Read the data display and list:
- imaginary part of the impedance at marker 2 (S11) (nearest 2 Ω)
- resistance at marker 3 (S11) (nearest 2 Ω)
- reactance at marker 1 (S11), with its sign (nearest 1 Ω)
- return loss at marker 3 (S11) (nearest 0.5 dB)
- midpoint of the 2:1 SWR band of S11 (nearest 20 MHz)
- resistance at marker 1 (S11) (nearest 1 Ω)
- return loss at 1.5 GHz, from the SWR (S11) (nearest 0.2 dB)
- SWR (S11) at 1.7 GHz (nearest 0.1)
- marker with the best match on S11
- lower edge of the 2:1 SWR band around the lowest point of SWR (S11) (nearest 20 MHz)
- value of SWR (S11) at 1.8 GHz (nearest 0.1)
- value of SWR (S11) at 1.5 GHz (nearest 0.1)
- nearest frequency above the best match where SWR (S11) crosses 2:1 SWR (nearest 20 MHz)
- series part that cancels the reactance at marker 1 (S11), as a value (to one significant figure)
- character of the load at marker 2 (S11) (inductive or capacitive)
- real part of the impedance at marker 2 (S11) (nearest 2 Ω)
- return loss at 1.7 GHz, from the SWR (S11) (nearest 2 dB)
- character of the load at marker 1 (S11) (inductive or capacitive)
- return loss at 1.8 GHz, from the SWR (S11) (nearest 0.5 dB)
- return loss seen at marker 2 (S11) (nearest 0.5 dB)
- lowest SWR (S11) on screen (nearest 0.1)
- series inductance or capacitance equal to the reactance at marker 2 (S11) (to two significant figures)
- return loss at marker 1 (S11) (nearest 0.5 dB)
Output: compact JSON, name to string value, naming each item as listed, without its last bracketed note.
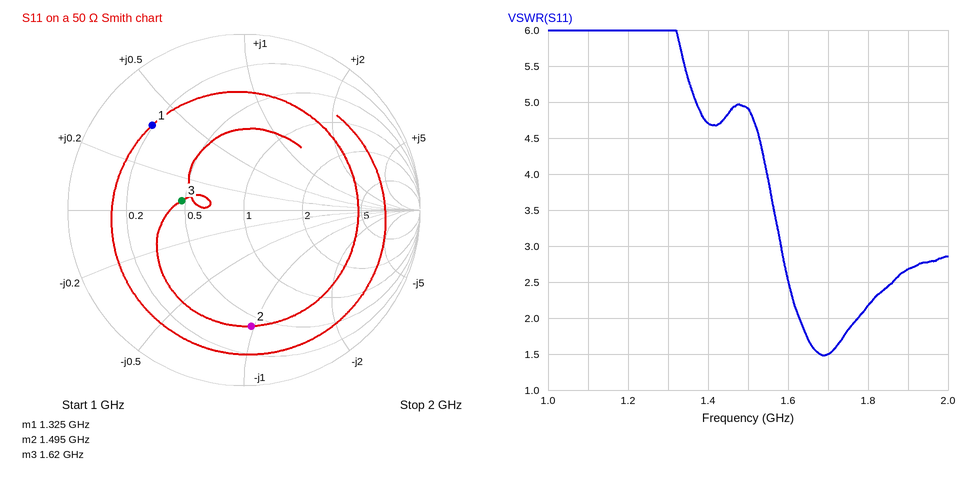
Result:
{"imaginary part of the impedance at marker 2 (S11)": "-48 Ω", "resistance at marker 3 (S11)": "24 Ω", "reactance at marker 1 (S11), with its sign": "+19 Ω", "return loss at marker 3 (S11)": "9.0 dB", "midpoint of the 2:1 SWR band of S11": "1.70 GHz", "resistance at marker 1 (S11)": "10 Ω", "return loss at 1.5 GHz, from the SWR (S11)": "3.6 dB", "SWR (S11) at 1.7 GHz": "1.5", "marker with the best match on S11": "marker 3", "lower edge of the 2:1 SWR band around the lowest point of SWR (S11)": "1.62 GHz", "value of SWR (S11) at 1.8 GHz": "2.2", "value of SWR (S11) at 1.5 GHz": "4.9", "nearest frequency above the best match where SWR (S11) crosses 2:1 SWR": "1.78 GHz", "series part that cancels the reactance at marker 1 (S11), as a value": "6 pF", "character of the load at marker 2 (S11)": "capacitive", "real part of the impedance at marker 2 (S11)": "20 Ω", "return loss at 1.7 GHz, from the SWR (S11)": "14 dB", "character of the load at marker 1 (S11)": "inductive", "return loss at 1.8 GHz, from the SWR (S11)": "8.5 dB", "return loss seen at marker 2 (S11)": "3.5 dB", "lowest SWR (S11) on screen": "1.5", "series inductance or capacitance equal to the reactance at marker 2 (S11)": "2.2 pF", "return loss at marker 1 (S11)": "3.0 dB"}
